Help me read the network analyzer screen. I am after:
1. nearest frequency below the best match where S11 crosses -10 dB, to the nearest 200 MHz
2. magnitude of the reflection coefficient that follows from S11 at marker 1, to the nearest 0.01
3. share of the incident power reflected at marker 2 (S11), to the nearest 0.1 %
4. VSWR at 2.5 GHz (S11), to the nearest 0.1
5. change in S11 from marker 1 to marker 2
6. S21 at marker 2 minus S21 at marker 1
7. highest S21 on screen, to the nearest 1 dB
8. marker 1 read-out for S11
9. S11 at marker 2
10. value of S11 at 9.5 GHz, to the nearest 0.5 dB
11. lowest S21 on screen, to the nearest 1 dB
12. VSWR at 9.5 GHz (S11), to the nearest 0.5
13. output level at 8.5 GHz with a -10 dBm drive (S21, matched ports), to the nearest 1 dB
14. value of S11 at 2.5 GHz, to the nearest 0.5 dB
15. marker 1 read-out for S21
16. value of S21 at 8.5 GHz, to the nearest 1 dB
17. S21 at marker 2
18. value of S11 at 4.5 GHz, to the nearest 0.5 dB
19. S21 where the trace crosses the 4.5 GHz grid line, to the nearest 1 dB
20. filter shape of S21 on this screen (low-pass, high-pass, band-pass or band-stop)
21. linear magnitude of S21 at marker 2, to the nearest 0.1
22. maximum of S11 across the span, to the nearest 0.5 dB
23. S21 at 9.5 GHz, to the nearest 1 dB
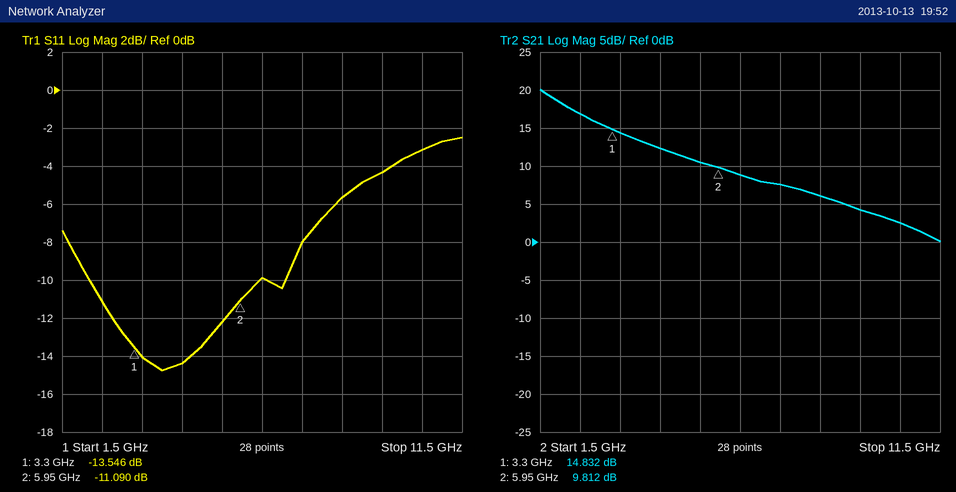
2.2 GHz
0.21
7.8 %
1.8
2.456 dB
-5.020 dB
20 dB
-13.546 dB
-11.090 dB
-4.5 dB
0 dB
4.0
-4 dBm
-11.0 dB
14.832 dB
6 dB
9.812 dB
-14.5 dB
12 dB
low-pass
3.1
-2.5 dB
4 dB
